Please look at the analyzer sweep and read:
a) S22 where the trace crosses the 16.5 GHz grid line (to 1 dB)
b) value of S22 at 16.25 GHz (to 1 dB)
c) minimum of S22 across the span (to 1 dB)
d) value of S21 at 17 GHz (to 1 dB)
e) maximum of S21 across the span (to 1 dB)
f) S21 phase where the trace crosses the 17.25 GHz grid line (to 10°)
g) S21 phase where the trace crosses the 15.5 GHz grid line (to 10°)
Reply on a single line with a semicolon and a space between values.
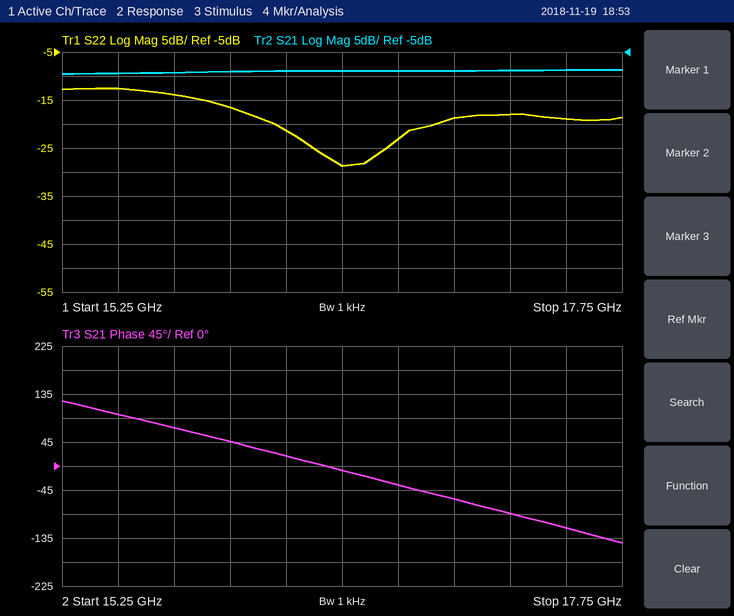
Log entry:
-29 dB; -21 dB; -29 dB; -9 dB; -9 dB; -90°; 100°
